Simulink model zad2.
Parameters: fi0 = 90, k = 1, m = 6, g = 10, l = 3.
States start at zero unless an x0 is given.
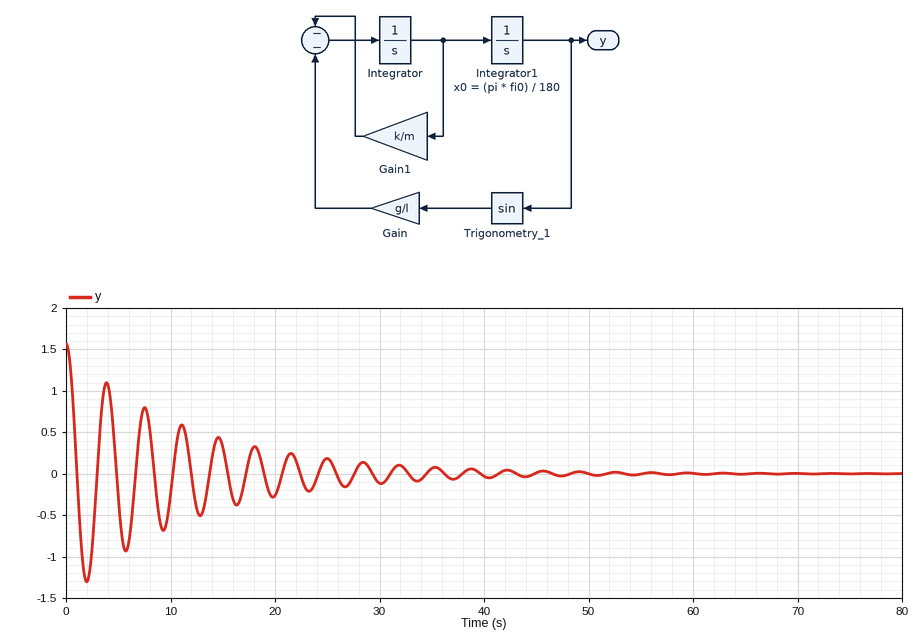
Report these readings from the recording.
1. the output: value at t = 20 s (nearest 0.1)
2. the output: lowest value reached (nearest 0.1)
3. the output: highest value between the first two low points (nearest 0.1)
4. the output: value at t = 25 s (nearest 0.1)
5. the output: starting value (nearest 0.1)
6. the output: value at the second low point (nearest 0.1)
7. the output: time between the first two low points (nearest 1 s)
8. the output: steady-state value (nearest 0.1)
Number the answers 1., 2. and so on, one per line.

1. -0.3
2. -1.3
3. 1.1
4. 0.2
5. 1.6
6. -0.9
7. 4 s
8. 0.0
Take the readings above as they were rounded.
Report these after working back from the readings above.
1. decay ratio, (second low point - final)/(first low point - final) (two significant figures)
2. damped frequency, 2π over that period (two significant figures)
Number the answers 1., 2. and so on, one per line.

1. 0.69
2. 1.6 rad/s
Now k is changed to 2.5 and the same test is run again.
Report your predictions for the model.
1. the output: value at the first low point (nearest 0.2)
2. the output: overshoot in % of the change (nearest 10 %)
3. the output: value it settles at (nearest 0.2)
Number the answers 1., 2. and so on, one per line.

1. -1.0
2. 60 %
3. 0.0
